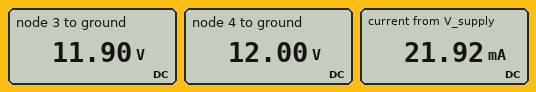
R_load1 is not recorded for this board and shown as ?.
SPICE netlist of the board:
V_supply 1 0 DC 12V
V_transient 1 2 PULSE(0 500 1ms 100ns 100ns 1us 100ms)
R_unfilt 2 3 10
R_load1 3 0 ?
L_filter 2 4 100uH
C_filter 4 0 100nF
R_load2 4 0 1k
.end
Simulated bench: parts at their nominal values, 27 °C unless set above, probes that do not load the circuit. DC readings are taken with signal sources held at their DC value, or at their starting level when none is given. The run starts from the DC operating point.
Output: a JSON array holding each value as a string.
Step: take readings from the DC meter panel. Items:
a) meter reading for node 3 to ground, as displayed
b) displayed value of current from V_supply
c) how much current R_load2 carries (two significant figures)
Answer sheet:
["11.90 V", "21.92 mA", "12 mA"]
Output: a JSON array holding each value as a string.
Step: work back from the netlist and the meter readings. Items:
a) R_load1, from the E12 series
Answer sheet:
["1.2 kΩ"]
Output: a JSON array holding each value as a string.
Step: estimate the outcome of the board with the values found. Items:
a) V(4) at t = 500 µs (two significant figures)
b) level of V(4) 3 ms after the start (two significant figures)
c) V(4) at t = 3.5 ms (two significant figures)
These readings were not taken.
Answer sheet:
["12 V", "12 V", "12 V"]
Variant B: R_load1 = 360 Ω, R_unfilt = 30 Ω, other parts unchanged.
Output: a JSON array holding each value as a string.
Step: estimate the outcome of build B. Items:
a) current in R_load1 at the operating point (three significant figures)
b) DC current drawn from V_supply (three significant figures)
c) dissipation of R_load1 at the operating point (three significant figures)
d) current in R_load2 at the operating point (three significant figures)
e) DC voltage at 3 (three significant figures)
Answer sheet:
["30.8 mA", "42.8 mA", "341 mW", "12.0 mA", "11.1 V"]
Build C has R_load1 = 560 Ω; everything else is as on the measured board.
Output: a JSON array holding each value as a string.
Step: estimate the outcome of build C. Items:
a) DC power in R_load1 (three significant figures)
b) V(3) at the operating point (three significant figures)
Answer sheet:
["248 mW", "11.8 V"]
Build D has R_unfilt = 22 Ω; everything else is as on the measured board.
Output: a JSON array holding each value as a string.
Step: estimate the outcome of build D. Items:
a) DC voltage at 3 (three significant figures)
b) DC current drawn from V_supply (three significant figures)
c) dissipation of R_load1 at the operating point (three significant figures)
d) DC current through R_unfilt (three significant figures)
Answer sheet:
["11.8 V", "21.8 mA", "116 mW", "9.82 mA"]
